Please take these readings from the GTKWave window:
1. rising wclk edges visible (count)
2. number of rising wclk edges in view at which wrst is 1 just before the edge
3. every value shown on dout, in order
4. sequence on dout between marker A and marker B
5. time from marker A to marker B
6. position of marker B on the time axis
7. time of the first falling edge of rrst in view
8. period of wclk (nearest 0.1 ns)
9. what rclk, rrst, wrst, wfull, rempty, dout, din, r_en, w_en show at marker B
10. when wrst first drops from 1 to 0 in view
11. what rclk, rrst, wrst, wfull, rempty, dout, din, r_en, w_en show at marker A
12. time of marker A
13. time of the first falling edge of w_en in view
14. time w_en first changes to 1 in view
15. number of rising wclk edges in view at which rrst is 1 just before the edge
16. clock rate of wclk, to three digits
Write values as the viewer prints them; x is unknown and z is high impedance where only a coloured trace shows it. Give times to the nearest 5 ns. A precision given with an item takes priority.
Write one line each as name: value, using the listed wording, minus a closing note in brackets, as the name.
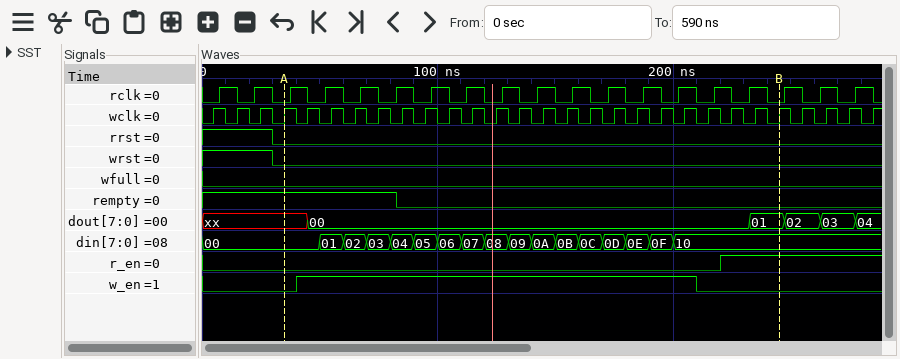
rising wclk edges visible: 29
number of rising wclk edges in view at which wrst is 1 just before the edge: 3
every value shown on dout, in order: xx, 00, 01, 02, 03, 04
sequence on dout between marker A and marker B: xx, 00, 01
time from marker A to marker B: 210 ns
position of marker B on the time axis: 245 ns
time of the first falling edge of rrst in view: 30 ns
period of wclk: 10 ns
what rclk, rrst, wrst, wfull, rempty, dout, din, r_en, w_en show at marker B: rclk=0, rrst=0, wrst=0, wfull=0, rempty=0, dout=01, din=10, r_en=1, w_en=0
when wrst first drops from 1 to 0 in view: 30 ns
what rclk, rrst, wrst, wfull, rempty, dout, din, r_en, w_en show at marker A: rclk=0, rrst=0, wrst=0, wfull=0, rempty=1, dout=xx, din=00, r_en=0, w_en=0
time of marker A: 35 ns
time of the first falling edge of w_en in view: 210 ns
time w_en first changes to 1 in view: 40 ns
number of rising wclk edges in view at which rrst is 1 just before the edge: 3
clock rate of wclk, to three digits: 100 MHz
